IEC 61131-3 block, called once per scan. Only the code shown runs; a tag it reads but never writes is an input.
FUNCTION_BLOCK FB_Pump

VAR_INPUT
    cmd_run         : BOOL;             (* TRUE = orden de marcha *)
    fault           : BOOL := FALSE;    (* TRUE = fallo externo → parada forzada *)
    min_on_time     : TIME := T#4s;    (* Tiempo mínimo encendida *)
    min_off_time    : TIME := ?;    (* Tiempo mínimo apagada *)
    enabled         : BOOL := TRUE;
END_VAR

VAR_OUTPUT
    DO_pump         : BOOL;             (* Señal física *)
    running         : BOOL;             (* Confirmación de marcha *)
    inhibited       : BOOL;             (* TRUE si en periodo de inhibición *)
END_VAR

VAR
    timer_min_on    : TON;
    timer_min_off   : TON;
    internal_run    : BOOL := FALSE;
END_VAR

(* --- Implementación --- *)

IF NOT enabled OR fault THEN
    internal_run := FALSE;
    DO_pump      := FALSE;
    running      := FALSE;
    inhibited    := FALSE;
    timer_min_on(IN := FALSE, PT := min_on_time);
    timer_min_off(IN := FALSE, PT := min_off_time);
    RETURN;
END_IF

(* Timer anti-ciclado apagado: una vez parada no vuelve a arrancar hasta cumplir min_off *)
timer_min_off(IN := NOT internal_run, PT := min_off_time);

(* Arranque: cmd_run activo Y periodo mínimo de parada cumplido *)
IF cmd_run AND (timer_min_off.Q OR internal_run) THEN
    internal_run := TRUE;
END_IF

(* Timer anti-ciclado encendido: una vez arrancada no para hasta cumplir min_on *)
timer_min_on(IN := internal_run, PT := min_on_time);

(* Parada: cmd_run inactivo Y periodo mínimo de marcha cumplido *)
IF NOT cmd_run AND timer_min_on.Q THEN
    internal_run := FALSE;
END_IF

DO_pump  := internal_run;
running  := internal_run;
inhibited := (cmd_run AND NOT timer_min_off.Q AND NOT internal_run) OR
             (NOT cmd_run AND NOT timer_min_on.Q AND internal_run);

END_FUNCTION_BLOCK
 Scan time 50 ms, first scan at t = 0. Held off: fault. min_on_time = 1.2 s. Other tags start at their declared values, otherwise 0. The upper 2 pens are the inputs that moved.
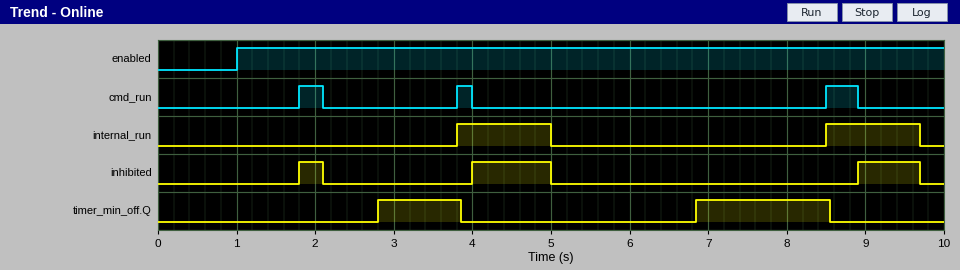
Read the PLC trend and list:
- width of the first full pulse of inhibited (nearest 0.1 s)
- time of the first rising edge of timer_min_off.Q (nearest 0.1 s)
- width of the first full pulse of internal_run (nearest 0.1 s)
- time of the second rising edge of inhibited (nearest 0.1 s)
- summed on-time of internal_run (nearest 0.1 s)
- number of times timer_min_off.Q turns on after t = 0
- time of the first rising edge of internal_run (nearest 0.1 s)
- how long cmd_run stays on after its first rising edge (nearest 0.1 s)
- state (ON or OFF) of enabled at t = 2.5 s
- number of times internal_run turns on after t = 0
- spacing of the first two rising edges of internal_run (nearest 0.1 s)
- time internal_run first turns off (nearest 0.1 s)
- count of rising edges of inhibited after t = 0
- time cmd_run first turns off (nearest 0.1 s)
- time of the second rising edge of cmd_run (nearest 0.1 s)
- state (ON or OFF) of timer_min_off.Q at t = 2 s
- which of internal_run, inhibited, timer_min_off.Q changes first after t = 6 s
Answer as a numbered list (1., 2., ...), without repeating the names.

1. 0.3 s
2. 2.8 s
3. 1.2 s
4. 4.0 s
5. 2.4 s
6. 2
7. 3.8 s
8. 0.3 s
9. ON
10. 2
11. 4.7 s
12. 5.0 s
13. 3
14. 2.1 s
15. 3.8 s
16. OFF
17. timer_min_off.Q
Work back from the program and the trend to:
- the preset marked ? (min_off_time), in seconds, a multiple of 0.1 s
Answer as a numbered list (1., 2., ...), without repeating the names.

1. 1.8 s
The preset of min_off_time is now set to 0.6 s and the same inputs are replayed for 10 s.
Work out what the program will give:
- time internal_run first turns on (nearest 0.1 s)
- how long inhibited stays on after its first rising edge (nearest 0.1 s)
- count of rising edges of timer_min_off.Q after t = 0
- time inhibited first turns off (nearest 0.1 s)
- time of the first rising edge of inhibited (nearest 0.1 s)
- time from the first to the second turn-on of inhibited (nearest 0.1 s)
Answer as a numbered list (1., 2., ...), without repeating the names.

1. 1.8 s
2. 0.9 s
3. 3
4. 3.0 s
5. 2.1 s
6. 1.9 s
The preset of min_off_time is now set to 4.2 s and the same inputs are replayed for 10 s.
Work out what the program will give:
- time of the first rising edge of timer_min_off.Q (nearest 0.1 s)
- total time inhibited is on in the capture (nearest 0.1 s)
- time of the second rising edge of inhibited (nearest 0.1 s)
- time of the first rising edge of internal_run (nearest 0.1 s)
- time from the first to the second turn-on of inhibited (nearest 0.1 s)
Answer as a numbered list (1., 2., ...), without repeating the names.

1. 5.2 s
2. 1.3 s
3. 3.8 s
4. 8.5 s
5. 2.0 s
